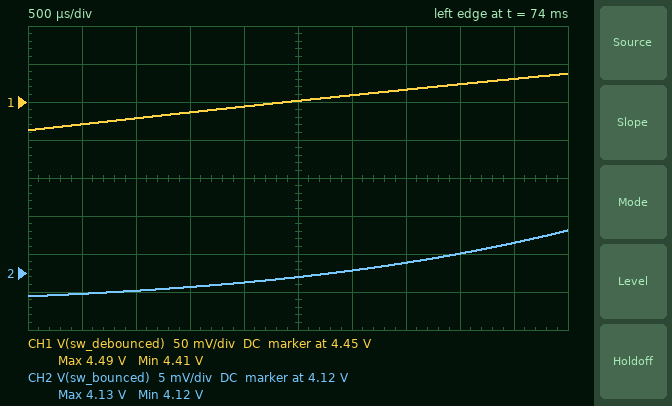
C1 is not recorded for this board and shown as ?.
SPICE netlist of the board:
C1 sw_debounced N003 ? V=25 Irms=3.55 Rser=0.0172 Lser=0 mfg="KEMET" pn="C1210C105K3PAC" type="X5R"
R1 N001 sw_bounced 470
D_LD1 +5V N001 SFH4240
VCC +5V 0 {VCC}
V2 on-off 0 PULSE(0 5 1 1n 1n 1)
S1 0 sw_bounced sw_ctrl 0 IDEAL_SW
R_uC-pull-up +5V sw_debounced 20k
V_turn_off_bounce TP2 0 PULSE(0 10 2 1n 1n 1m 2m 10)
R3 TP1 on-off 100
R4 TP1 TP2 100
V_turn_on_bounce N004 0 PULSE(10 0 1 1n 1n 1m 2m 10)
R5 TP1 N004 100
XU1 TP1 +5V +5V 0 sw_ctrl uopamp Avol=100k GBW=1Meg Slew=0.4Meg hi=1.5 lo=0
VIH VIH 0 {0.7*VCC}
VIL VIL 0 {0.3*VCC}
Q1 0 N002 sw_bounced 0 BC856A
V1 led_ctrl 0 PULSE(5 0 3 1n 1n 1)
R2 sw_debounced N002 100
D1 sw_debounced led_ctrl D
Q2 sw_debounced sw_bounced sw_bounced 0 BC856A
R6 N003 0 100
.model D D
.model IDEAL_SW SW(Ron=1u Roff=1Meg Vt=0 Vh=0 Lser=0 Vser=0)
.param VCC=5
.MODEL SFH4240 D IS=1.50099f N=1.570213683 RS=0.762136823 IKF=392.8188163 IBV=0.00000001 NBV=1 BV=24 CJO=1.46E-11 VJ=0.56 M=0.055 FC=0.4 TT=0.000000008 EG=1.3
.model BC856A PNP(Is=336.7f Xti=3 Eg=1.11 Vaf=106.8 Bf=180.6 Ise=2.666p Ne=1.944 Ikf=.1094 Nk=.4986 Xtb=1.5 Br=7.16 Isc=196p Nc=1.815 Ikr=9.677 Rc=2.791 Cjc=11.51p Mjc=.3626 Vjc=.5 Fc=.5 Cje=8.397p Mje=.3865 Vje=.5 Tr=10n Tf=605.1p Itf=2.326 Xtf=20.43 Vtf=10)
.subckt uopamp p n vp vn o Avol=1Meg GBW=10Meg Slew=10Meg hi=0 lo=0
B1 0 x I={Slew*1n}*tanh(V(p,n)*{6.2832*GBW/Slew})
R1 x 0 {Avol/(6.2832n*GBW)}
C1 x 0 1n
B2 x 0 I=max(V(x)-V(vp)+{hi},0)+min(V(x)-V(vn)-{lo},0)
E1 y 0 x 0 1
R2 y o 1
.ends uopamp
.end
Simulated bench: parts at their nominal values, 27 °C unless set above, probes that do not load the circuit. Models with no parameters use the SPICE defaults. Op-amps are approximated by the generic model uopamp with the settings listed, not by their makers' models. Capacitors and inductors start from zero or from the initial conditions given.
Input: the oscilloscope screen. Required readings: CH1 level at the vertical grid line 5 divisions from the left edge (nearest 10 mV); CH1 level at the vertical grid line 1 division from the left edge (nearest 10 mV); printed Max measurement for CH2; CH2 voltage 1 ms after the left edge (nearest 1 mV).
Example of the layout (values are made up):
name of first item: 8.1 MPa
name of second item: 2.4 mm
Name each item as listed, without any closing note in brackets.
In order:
CH1 level at the vertical grid line 5 divisions from the left edge: 4.45 V
CH1 level at the vertical grid line 1 division from the left edge: 4.42 V
printed Max measurement for CH2: 4.13 V
CH2 voltage 1 ms after the left edge: 4.118 V
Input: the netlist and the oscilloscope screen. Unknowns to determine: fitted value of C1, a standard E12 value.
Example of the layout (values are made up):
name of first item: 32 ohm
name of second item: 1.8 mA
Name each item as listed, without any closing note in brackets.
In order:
fitted value of C1, a standard E12 value: 1.8 µF
